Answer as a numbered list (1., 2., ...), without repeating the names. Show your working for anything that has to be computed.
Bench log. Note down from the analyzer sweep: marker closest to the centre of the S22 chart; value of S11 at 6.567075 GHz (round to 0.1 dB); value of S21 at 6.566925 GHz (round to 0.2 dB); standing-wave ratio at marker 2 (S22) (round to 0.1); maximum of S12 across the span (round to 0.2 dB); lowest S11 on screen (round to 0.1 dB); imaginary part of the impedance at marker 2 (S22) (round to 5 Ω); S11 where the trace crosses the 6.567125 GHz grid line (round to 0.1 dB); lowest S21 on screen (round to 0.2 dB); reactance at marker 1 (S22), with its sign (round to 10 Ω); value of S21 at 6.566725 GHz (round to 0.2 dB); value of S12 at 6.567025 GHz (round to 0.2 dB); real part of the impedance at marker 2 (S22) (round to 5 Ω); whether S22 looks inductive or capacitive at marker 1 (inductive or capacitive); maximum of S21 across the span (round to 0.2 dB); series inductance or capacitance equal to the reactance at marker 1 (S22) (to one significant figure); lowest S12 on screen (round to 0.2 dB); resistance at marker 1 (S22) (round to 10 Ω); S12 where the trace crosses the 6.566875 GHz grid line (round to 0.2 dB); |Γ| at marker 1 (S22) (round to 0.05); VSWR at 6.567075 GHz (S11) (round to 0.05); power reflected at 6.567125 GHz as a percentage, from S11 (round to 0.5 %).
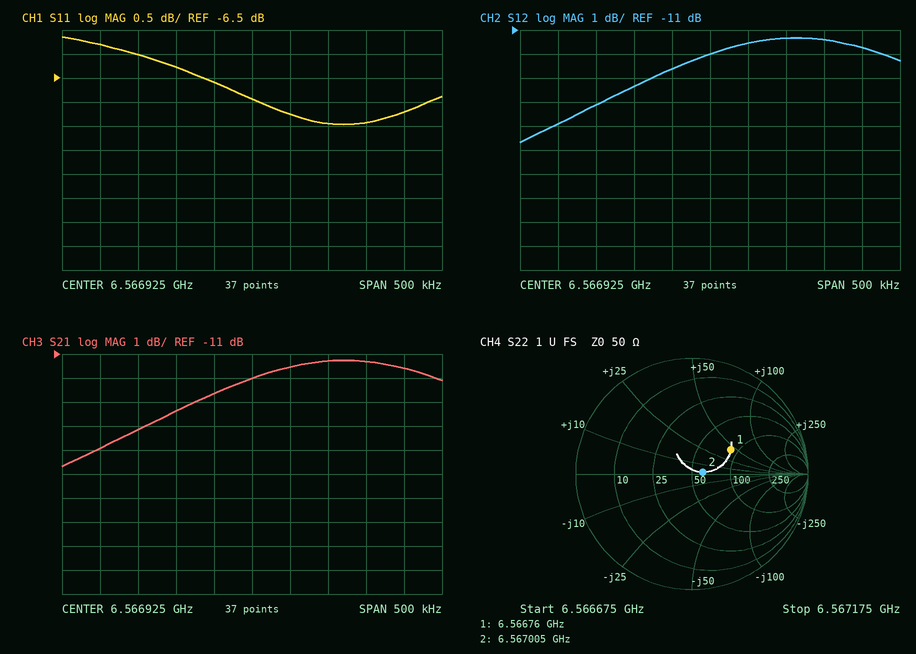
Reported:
1. marker 2
2. -7.4 dB
3. -12.0 dB
4. 1.2
5. -11.4 dB
6. -7.5 dB
7. 0 Ω
8. -7.2 dB
9. -15.6 dB
10. +40 Ω
11. -15.0 dB
12. -11.4 dB
13. 60 Ω
14. inductive
15. -11.2 dB
16. L = 40 Ω/(2π × 6.56676 GHz) ≈ 1 nH
17. -15.6 dB
18. 90 Ω
19. -12.6 dB
20. 0.40
21. |Γ| = 10^(-7.4/20) = 0.4266; VSWR = (1 + 0.4266)/(1 − 0.4266) ≈ 2.49, so 2.50 to the nearest 0.05
22. 10^(-7.2/10) ≈ 19.1 %, so 19.0 % to the nearest 0.5 %
